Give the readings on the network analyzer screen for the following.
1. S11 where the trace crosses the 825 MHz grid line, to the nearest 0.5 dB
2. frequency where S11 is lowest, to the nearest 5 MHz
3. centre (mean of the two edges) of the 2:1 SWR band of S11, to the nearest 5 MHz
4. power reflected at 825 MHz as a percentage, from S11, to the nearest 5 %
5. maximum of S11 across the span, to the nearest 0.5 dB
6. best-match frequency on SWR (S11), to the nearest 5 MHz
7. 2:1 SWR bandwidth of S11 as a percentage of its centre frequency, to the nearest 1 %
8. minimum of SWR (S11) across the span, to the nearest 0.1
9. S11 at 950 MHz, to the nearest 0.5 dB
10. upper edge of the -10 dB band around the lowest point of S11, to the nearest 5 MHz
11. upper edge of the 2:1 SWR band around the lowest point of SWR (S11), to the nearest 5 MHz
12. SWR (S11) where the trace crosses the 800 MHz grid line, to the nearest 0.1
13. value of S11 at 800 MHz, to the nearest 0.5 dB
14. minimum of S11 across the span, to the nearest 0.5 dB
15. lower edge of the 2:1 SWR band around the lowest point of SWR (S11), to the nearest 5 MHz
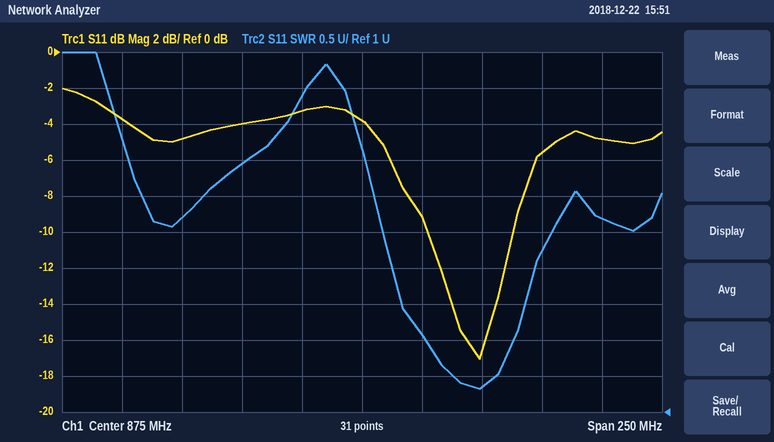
-4.0 dB
925 MHz
920 MHz
40 %
-2.0 dB
925 MHz
4 %
1.3
-5.5 dB
940 MHz
940 MHz
3.7
-5.0 dB
-17.0 dB
900 MHz
